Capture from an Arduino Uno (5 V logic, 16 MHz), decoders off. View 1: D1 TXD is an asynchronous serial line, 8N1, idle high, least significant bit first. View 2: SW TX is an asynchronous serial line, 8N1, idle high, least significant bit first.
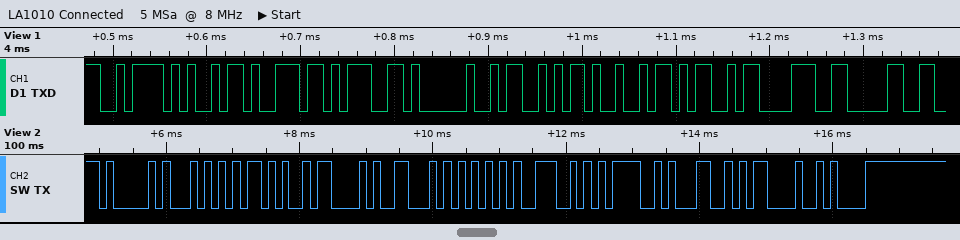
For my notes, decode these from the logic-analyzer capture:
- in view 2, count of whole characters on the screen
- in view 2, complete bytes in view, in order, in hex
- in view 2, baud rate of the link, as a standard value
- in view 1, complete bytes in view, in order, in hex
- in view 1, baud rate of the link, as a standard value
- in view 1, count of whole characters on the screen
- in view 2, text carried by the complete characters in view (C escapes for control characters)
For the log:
11
0x41 0x54 0x2B 0x43 0x46 0x55 0x4E 0x3D 0x31 0x0D 0x0A
9600 baud
0x7A 0x69 0x6E 0x67 0x20 0x53 0x49 0x4D 0x38 0x30
115200 baud
10
"AT+CFUN=1\r\n"
